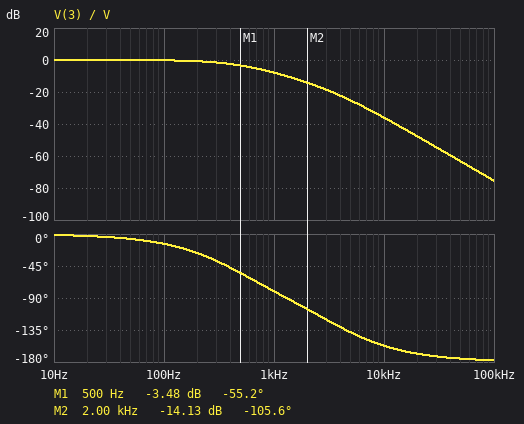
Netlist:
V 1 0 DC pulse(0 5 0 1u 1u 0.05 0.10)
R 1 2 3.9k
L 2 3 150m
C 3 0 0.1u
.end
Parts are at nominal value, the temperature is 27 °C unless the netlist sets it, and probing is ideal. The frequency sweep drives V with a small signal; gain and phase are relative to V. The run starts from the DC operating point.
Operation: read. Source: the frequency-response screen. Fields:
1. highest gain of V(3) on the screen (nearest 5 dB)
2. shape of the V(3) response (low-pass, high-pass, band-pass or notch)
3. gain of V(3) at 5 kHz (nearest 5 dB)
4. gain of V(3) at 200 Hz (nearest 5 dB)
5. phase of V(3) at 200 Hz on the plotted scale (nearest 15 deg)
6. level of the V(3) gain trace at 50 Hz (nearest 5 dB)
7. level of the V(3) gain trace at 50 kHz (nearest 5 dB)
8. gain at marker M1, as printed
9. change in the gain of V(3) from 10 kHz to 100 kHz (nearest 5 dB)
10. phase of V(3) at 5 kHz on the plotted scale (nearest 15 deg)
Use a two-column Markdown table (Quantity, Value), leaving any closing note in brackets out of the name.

| Quantity | Value |
|---|---|
| highest gain of V(3) on the screen | 0 dB |
| shape of the V(3) response | low-pass |
| gain of V(3) at 5 kHz | -25 dB |
| gain of V(3) at 200 Hz | 0 dB |
| phase of V(3) at 200 Hz on the plotted scale | -30 deg |
| level of the V(3) gain trace at 50 Hz | 0 dB |
| level of the V(3) gain trace at 50 kHz | -65 dB |
| gain at marker M1, as printed | -3.48 dB |
| change in the gain of V(3) from 10 kHz to 100 kHz | -40 dB |
| phase of V(3) at 5 kHz on the plotted scale | -135 deg |
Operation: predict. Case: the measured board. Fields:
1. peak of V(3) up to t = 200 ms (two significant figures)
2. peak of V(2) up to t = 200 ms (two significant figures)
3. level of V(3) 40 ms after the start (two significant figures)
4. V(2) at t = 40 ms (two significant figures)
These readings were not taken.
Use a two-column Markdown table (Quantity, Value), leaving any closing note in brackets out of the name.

| Quantity | Value |
|---|---|
| peak of V(3) up to t = 200 ms | 5.0 V |
| peak of V(2) up to t = 200 ms | 5.0 V |
| level of V(3) 40 ms after the start | 5.0 V |
| V(2) at t = 40 ms | 5.0 V |
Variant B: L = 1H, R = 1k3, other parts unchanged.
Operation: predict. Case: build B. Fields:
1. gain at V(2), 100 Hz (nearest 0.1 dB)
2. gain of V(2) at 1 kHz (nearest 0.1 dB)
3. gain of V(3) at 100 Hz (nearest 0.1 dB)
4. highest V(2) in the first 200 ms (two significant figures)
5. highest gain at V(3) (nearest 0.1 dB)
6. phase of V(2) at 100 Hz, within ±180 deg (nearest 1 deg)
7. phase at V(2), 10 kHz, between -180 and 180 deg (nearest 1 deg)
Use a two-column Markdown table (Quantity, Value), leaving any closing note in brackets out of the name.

| Quantity | Value |
|---|---|
| gain at V(2), 100 Hz | 0 dB |
| gain of V(2) at 1 kHz | -0.3 dB |
| gain of V(3) at 100 Hz | 0.3 dB |
| highest V(2) in the first 200 ms | 5.8 V |
| highest gain at V(3) | 7.9 dB |
| phase of V(2) at 100 Hz, within ±180 deg | -5 deg |
| phase at V(2), 10 kHz, between -180 and 180 deg | 1 deg |
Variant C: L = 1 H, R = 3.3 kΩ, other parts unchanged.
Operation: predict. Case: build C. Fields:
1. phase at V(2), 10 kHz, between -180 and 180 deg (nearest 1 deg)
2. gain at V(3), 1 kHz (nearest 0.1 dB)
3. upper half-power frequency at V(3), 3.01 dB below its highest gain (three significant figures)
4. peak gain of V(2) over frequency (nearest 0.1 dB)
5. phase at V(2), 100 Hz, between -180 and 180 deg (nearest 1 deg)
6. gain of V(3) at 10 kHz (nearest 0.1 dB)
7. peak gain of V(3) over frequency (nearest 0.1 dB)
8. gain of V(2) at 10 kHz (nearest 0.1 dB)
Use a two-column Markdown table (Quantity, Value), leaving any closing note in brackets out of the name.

| Quantity | Value |
|---|---|
| phase at V(2), 10 kHz, between -180 and 180 deg | 3 deg |
| gain at V(3), 1 kHz | -11.1 dB |
| upper half-power frequency at V(3), 3.01 dB below its highest gain | 584 Hz |
| peak gain of V(2) over frequency | 0 dB |
| phase at V(2), 100 Hz, between -180 and 180 deg | -12 deg |
| gain of V(3) at 10 kHz | -51.9 dB |
| peak gain of V(3) over frequency | 1.0 dB |
| gain of V(2) at 10 kHz | 0 dB |
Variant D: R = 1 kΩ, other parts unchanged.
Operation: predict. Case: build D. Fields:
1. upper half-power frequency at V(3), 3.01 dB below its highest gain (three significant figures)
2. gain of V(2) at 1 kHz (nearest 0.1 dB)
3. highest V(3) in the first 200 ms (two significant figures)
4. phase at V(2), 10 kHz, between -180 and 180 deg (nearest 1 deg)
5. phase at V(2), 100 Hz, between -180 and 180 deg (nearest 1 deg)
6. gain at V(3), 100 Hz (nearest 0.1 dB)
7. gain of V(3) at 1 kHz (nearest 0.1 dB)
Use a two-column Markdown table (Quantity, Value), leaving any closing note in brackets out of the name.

| Quantity | Value |
|---|---|
| upper half-power frequency at V(3), 3.01 dB below its highest gain | 1.54 kHz |
| gain of V(2) at 1 kHz | -5.3 dB |
| highest V(3) in the first 200 ms | 6.3 V |
| phase at V(2), 10 kHz, between -180 and 180 deg | 6 deg |
| phase at V(2), 100 Hz, between -180 and 180 deg | -4 deg |
| gain at V(3), 100 Hz | 0 dB |
| gain of V(3) at 1 kHz | 2.5 dB |
